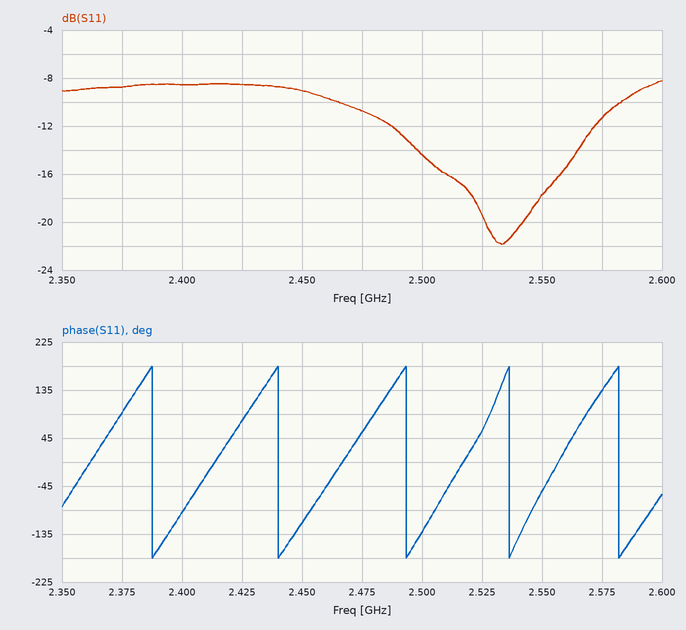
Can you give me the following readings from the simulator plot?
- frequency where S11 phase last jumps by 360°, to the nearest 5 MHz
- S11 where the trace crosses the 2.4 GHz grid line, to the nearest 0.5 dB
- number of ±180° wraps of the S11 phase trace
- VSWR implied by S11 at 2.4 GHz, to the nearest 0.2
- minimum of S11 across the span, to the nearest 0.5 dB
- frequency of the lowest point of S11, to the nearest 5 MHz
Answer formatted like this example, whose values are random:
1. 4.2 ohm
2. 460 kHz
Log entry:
1. 2.580 GHz
2. -8.5 dB
3. 5
4. 2.2
5. -22.0 dB
6. 2.535 GHz
